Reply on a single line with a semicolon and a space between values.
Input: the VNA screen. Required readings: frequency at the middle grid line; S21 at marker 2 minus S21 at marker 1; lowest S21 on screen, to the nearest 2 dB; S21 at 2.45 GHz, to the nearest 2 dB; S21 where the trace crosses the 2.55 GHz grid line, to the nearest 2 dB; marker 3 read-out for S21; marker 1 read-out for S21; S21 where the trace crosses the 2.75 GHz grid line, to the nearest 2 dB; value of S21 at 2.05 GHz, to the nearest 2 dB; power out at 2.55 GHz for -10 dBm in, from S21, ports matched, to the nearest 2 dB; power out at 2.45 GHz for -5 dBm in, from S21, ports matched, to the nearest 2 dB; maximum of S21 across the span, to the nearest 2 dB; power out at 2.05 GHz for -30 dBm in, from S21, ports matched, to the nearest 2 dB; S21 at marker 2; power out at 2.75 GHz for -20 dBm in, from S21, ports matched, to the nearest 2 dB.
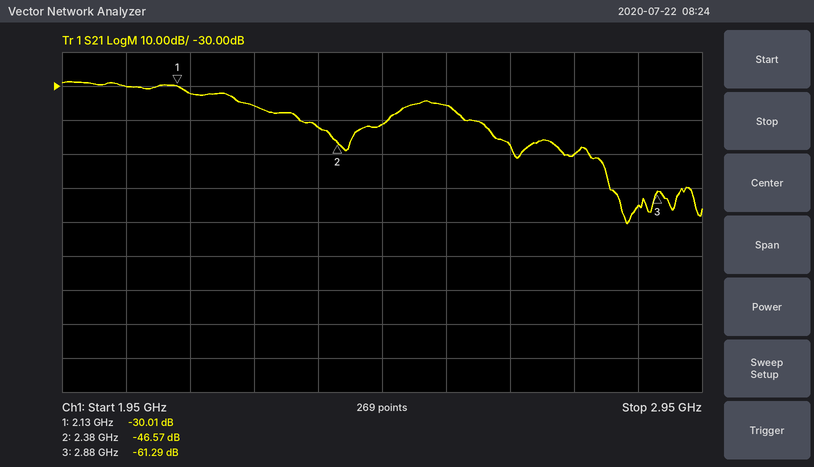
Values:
2.45 GHz; -16.56 dB; -70 dB; -42 dB; -36 dB; -61.29 dB; -30.01 dB; -50 dB; -30 dB; -46 dBm; -46 dBm; -28 dB; -60 dBm; -46.57 dB; -70 dBm
